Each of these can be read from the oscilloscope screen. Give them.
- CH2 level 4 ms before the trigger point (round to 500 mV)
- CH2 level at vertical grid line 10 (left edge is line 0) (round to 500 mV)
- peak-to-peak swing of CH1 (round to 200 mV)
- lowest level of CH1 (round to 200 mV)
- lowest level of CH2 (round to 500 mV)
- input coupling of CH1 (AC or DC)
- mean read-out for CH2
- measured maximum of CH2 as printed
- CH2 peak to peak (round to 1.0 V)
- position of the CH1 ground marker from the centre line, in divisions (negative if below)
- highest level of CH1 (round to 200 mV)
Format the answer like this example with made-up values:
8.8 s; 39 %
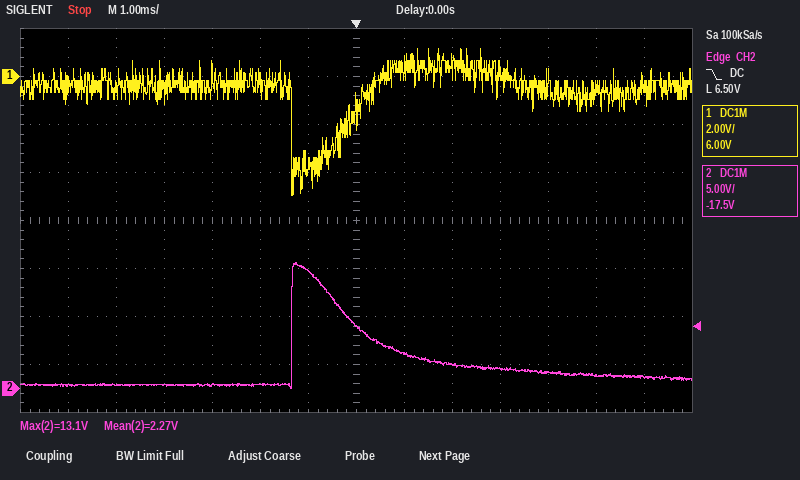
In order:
500 mV; 2.0 V; 6.2 V; -5.0 V; 0.0 V; DC; 2.27 V; 13.1 V; 13.0 V; +3.0 div; 1.2 V
